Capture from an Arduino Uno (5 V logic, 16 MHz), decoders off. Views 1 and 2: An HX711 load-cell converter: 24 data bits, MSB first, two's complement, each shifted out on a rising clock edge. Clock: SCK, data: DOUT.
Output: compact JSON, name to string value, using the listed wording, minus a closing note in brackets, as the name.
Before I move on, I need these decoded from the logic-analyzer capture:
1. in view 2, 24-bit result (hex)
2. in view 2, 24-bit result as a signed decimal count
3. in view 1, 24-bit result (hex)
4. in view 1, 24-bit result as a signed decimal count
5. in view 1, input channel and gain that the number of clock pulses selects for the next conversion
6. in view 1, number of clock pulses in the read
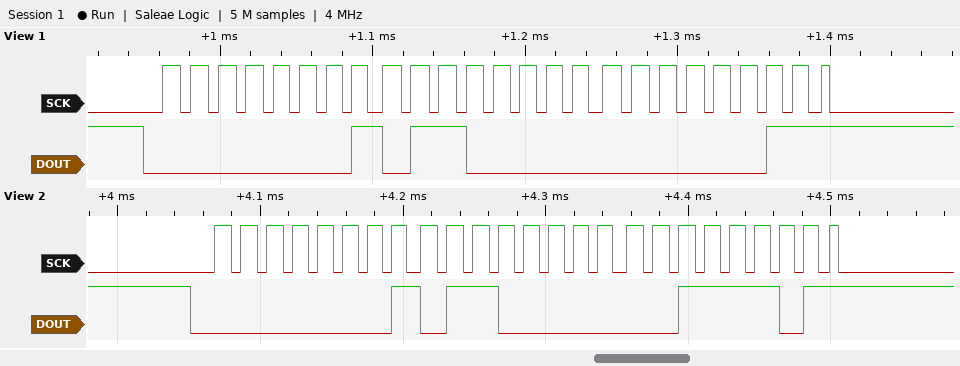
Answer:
{"in view 2, 24-bit result": "0x01603D", "in view 2, 24-bit result as a signed decimal count": "90173", "in view 1, 24-bit result": "0x016003", "in view 1, 24-bit result as a signed decimal count": "90115", "in view 1, input channel and gain that the number of clock pulses selects for the next conversion": "channel A, gain 128", "in view 1, number of clock pulses in the read": "25"}
